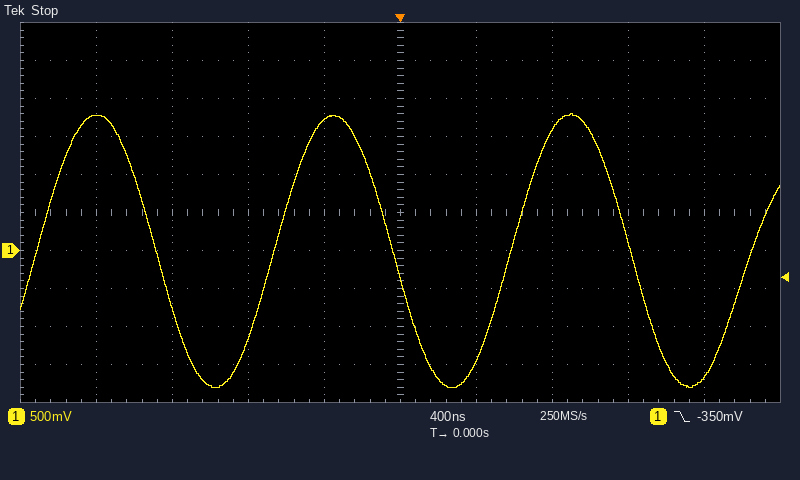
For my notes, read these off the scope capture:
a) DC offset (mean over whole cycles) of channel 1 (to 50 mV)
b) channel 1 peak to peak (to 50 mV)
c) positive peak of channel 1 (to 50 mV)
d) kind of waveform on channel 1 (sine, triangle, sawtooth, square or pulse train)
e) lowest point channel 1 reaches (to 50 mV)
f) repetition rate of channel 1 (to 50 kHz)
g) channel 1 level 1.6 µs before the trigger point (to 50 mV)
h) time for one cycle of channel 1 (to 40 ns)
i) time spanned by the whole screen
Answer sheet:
0 mV
3.60 V
1.80 V
sine
-1.80 V
800 kHz
1.80 V
1.24 µs
4 µs
